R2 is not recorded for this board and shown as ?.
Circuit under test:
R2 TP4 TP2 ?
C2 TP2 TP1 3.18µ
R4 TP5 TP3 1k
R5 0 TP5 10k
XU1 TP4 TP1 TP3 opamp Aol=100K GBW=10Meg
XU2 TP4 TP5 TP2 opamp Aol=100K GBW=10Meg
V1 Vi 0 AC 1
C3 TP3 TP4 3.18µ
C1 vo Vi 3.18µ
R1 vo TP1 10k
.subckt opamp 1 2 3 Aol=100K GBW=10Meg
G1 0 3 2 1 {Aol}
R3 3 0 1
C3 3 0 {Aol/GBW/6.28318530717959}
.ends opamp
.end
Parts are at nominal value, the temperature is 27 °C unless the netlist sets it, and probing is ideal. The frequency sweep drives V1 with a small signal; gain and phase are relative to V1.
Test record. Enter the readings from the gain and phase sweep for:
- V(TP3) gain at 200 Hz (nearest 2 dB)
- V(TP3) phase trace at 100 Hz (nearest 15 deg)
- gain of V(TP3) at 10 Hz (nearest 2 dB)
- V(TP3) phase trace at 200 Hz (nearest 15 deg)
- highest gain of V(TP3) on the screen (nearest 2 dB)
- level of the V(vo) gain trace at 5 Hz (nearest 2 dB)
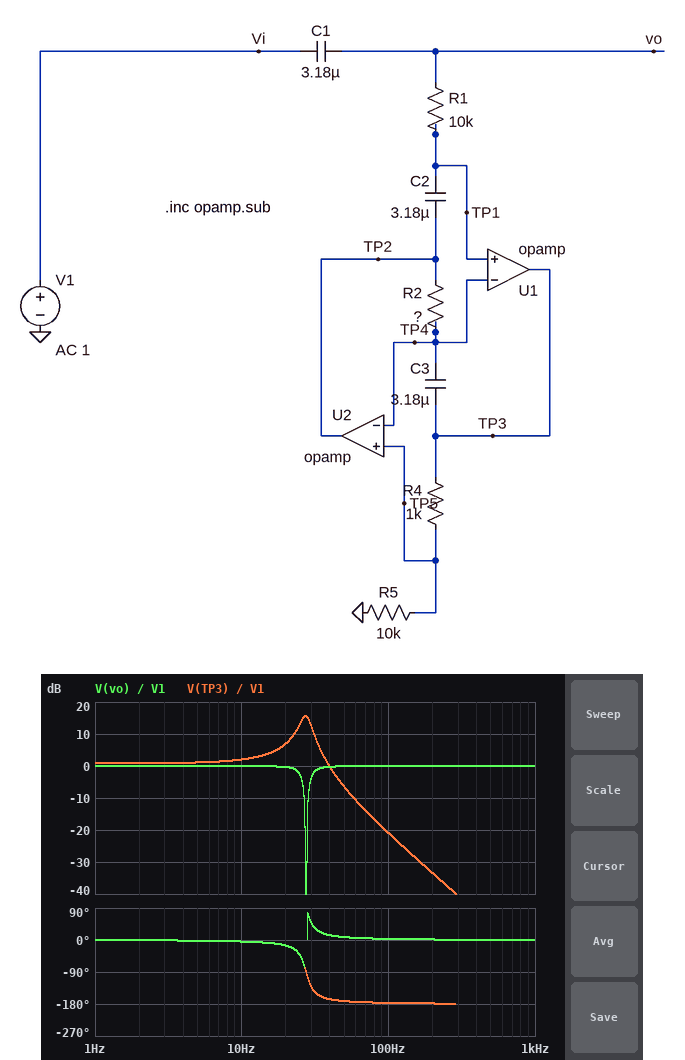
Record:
-34 dB
-180 deg
2 dB
-180 deg
16 dB
0 dB
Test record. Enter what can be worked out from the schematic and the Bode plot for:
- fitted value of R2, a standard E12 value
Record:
3.3 kΩ
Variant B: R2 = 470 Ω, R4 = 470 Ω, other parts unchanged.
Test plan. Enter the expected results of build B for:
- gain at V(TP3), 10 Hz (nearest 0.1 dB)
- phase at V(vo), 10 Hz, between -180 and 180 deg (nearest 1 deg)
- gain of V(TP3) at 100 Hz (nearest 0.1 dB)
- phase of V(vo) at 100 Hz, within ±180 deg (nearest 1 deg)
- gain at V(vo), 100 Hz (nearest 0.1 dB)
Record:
0.5 dB
0 deg
18.4 dB
-21 deg
-0.6 dB
